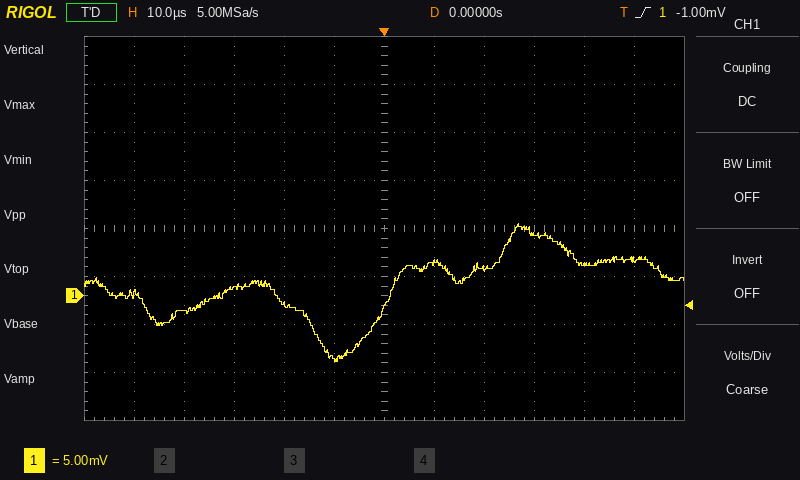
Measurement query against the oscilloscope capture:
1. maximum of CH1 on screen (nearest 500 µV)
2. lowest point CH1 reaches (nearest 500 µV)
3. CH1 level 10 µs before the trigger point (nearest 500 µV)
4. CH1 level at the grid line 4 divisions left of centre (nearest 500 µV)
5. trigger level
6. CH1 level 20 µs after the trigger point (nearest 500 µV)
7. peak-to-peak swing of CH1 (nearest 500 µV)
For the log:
7.5 mV
-7.0 mV
-6.5 mV
-1.5 mV
-1.00 mV
3.0 mV
14.5 mV
